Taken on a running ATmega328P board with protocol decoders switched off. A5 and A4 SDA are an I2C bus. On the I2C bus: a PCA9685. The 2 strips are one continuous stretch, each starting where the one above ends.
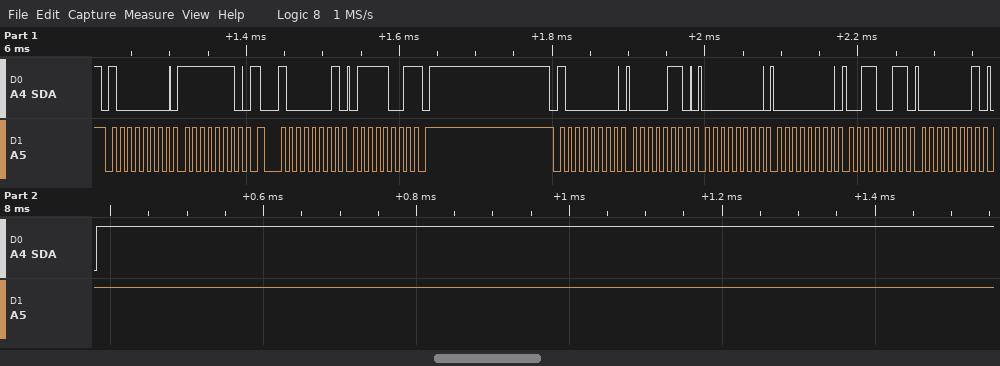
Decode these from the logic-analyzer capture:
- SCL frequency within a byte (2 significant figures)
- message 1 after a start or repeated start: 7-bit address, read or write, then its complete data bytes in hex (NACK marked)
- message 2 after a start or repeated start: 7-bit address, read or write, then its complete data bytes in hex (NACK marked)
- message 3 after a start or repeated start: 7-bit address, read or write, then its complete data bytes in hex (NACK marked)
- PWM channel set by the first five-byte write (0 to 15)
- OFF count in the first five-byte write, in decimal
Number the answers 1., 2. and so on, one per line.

1. 100 kHz
2. 0x40 write: FE
3. 0x40 read: 79 NACK
4. 0x40 write: 06 00 00 33 01
5. 0
6. 307
